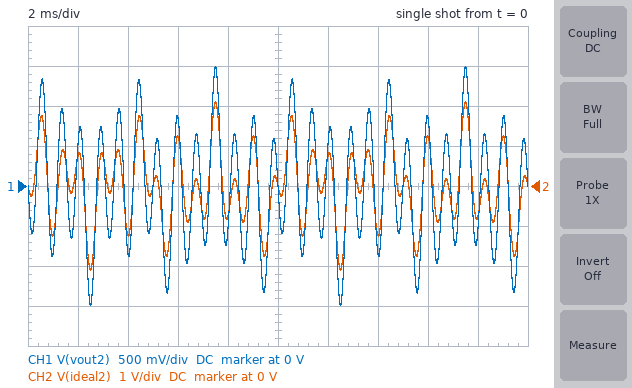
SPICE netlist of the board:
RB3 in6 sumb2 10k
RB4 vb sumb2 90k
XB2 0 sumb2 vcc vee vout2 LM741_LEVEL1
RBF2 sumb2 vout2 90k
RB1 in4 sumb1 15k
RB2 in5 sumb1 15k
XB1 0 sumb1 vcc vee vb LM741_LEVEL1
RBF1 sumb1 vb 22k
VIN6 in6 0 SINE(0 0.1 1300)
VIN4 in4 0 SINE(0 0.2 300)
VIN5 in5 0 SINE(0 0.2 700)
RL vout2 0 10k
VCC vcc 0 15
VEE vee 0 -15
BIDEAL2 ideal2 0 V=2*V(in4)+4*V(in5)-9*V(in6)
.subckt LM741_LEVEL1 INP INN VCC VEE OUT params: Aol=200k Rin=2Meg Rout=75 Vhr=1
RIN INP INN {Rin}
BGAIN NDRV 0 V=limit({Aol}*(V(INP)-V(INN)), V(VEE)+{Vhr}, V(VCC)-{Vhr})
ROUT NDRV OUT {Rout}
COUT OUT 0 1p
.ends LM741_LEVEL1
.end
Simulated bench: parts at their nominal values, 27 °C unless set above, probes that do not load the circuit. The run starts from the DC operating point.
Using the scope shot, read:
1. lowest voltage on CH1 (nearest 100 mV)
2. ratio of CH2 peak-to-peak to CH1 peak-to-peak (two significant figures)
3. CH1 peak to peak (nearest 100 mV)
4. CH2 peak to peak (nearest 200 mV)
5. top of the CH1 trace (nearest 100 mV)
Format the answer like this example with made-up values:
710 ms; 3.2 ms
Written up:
-1.5 V; 1.4; 3.0 V; 4.2 V; 1.5 V
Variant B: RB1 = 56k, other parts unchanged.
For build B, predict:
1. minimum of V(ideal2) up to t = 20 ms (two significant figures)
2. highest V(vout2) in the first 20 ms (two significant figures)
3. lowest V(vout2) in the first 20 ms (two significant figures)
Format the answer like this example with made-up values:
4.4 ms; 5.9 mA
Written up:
-2.1 V; 1.3 V; -1.3 V
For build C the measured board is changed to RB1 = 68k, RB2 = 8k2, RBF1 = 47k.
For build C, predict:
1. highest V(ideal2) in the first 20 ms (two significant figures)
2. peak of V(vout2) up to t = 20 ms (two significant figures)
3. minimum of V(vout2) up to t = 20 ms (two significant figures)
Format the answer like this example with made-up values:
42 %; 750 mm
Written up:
2.1 V; 2.2 V; -2.2 V
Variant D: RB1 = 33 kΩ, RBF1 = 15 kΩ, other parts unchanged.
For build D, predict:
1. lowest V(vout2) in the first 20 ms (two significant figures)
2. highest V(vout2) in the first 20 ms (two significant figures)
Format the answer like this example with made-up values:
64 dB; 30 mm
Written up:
-1.2 V; 1.2 V
